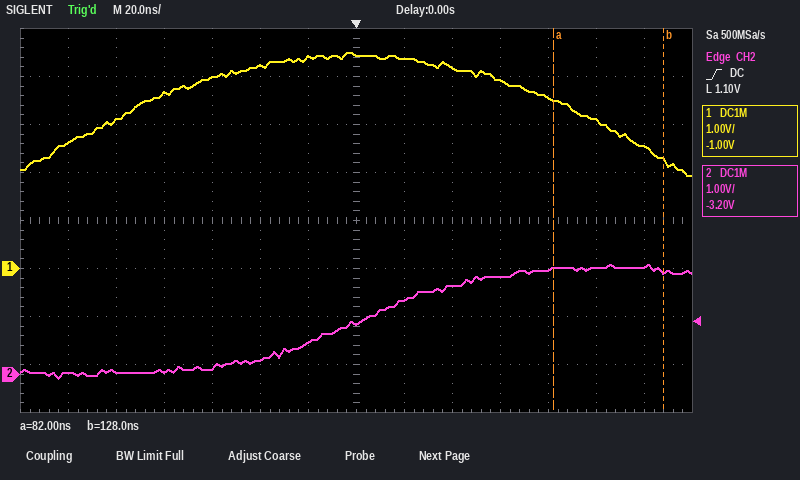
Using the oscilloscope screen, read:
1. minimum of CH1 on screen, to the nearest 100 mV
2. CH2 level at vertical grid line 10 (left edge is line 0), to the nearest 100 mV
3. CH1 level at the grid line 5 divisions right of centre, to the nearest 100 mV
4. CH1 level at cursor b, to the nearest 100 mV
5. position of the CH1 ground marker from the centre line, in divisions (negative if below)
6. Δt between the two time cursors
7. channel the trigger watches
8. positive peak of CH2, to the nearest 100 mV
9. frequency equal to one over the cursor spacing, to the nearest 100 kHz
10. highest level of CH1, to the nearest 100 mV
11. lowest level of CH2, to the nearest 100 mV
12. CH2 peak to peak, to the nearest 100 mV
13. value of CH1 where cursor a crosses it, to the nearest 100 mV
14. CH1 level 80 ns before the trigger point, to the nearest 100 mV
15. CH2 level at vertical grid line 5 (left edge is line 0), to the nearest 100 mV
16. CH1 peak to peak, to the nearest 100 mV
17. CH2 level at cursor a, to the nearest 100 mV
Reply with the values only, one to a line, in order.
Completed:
1.9 V
2.0 V
3.1 V
2.2 V
-1.0 div
46 ns
CH2
2.3 V
21.7 MHz
4.5 V
-100 mV
2.4 V
3.5 V
3.7 V
300 mV
2.6 V
2.2 V
